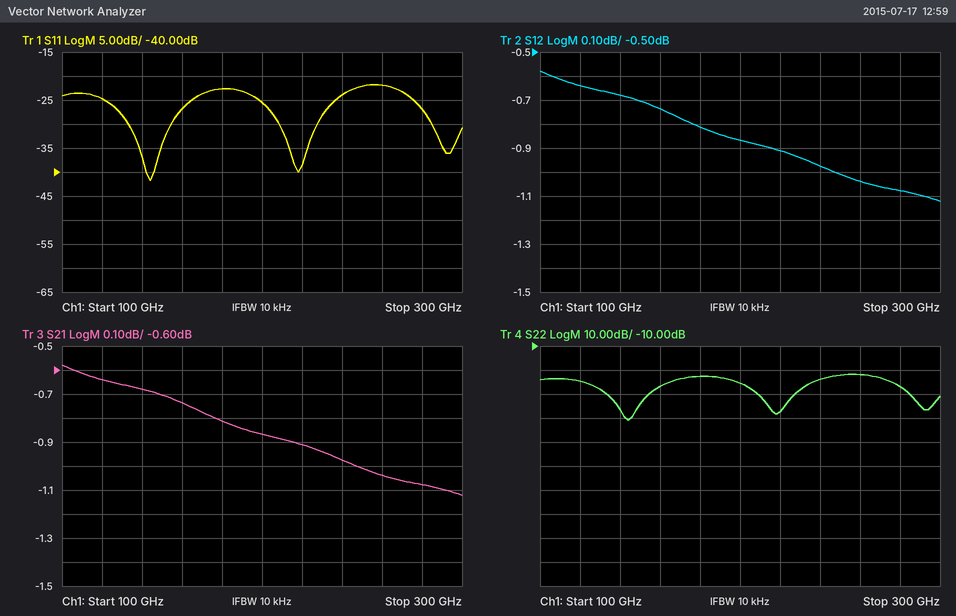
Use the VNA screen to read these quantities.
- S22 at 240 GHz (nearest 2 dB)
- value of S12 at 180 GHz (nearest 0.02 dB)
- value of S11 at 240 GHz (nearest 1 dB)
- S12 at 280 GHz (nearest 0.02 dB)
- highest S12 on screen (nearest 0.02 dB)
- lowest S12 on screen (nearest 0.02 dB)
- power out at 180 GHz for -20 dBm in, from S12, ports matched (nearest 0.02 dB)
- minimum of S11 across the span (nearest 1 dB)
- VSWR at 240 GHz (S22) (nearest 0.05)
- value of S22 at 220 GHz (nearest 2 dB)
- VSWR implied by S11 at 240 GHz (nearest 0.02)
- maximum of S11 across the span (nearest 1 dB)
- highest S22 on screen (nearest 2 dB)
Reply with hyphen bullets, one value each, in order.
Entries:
- -24 dB
- -0.82 dB
- -24 dB
- -1.08 dB
- -0.58 dB
- -1.12 dB
- -20.82 dBm
- -42 dB
- 1.15
- -38 dB
- 1.14
- -22 dB
- -22 dB
